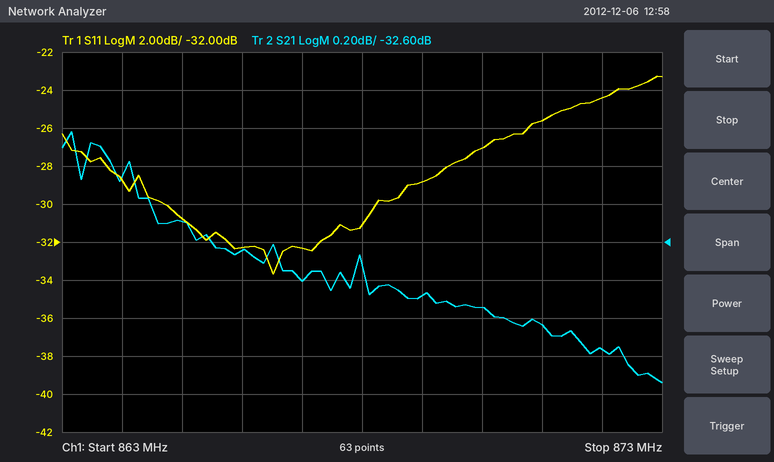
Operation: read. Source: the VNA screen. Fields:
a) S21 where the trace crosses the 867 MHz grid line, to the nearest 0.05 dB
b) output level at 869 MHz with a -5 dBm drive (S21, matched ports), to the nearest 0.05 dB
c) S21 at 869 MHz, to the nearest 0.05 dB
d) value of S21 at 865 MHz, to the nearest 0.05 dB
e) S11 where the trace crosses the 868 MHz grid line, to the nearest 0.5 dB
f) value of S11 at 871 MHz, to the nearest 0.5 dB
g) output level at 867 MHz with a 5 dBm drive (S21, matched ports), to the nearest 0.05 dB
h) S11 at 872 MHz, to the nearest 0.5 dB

-32.80 dB
-37.90 dBm
-32.90 dB
-32.50 dB
-31.0 dB
-25.5 dB
-27.80 dBm
-24.5 dB
